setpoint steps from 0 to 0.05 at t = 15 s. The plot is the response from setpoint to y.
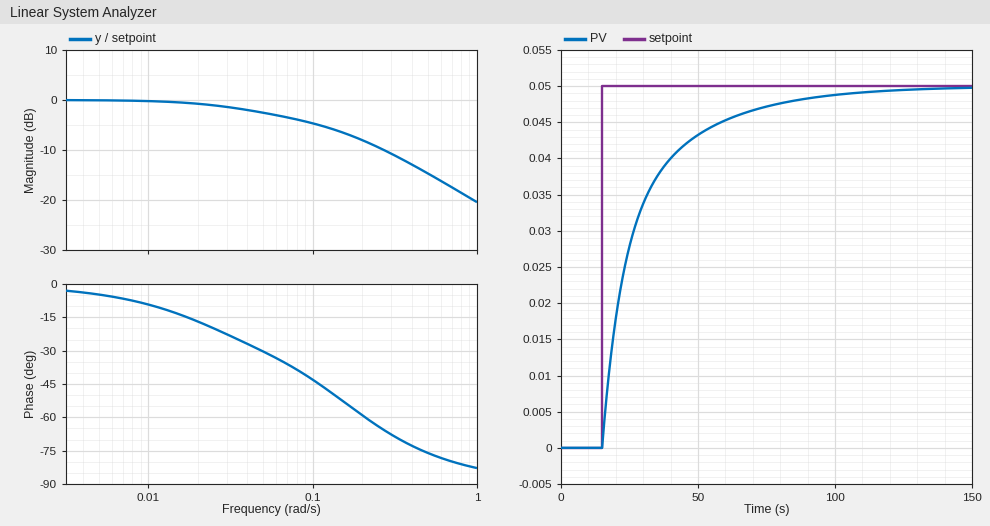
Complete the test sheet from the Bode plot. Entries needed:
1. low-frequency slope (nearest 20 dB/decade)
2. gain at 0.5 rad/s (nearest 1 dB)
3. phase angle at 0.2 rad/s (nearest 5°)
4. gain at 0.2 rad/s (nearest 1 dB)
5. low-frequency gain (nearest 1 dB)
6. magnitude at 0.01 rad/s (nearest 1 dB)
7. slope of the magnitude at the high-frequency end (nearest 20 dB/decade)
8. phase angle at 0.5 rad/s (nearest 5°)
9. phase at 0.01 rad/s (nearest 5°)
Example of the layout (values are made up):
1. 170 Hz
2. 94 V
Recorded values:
1. 0 dB/decade
2. -15 dB
3. -60°
4. -8 dB
5. 0 dB
6. 0 dB
7. -20 dB/decade
8. -75°
9. -10°
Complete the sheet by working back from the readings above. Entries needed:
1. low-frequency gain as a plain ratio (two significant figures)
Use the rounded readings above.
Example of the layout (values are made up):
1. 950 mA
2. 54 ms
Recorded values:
1. 1.0
